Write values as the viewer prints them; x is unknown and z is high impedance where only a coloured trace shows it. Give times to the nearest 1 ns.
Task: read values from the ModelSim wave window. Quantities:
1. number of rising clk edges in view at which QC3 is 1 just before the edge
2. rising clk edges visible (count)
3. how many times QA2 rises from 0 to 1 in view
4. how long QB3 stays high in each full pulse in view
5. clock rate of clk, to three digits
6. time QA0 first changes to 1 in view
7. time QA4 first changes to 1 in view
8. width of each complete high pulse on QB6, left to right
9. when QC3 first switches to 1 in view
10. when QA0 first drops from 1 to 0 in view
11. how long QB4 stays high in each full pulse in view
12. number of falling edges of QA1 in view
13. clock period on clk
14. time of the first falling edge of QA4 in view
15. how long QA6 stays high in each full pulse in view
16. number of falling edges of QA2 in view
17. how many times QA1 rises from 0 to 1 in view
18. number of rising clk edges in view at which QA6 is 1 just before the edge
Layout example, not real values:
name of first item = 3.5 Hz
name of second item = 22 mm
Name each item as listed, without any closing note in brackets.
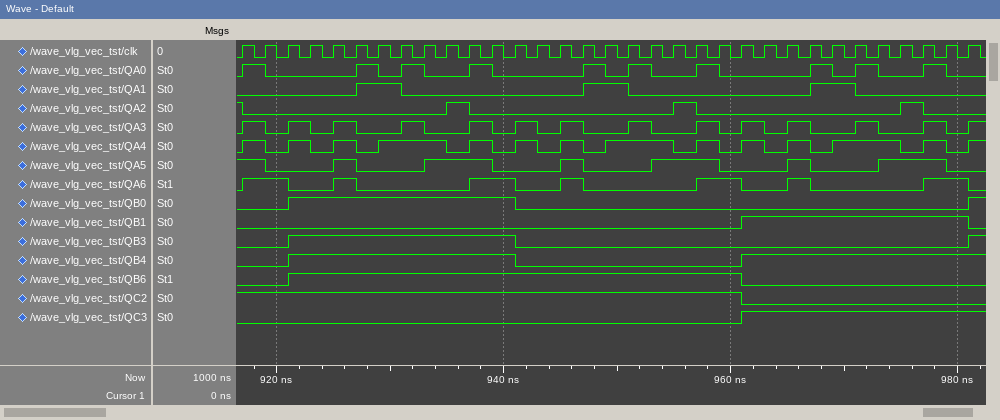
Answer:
number of rising clk edges in view at which QC3 is 1 just before the edge = 10
rising clk edges visible = 33
how many times QA2 rises from 0 to 1 in view = 3
how long QB3 stays high in each full pulse in view = 20 ns
clock rate of clk, to three digits = 500 MHz
time QA0 first changes to 1 in view = 917 ns
time QA4 first changes to 1 in view = 917 ns
width of each complete high pulse on QB6, left to right = 40 ns
when QC3 first switches to 1 in view = 961 ns
when QA0 first drops from 1 to 0 in view = 919 ns
how long QB4 stays high in each full pulse in view = 20 ns
number of falling edges of QA1 in view = 3
clock period on clk = 2 ns
time of the first falling edge of QA4 in view = 919 ns
how long QA6 stays high in each full pulse in view = 4 ns, 2 ns, 4 ns, 2 ns, 4 ns, 2 ns, 4 ns
number of falling edges of QA2 in view = 4
how many times QA1 rises from 0 to 1 in view = 3
number of rising clk edges in view at which QA6 is 1 just before the edge = 11
